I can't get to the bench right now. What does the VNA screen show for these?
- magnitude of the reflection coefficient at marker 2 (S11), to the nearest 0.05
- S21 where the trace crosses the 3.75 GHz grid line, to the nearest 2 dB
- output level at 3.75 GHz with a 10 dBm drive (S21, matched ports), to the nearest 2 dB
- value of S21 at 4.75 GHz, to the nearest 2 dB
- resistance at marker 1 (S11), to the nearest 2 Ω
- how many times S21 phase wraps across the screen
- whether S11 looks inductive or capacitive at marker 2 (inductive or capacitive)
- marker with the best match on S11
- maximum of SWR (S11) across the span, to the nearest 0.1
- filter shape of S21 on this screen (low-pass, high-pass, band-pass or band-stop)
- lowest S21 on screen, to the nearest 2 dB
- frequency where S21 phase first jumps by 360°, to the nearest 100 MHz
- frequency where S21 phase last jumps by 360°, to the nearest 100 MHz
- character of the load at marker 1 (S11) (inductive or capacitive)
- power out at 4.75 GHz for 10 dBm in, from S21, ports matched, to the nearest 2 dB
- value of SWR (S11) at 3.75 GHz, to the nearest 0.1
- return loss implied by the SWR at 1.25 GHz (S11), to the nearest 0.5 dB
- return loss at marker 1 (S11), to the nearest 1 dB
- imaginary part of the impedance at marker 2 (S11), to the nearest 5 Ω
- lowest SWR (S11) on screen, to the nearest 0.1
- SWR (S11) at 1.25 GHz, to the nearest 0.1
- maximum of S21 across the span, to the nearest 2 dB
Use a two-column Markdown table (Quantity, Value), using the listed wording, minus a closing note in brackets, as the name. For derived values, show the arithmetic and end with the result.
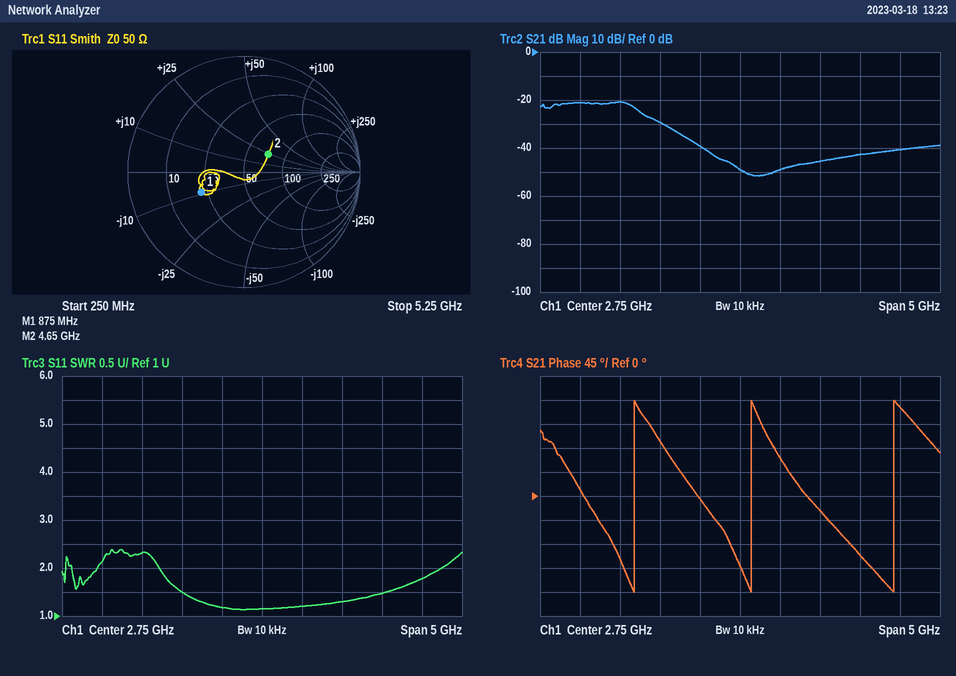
| Quantity | Value |
|---|---|
| magnitude of the reflection coefficient at marker 2 (S11), to the nearest 0.05 | 0.25 |
| S21 where the trace crosses the 3.75 GHz grid line, to the nearest 2 dB | -46 dB |
| output level at 3.75 GHz with a 10 dBm drive (S21, matched ports), to the nearest 2 dB | 10 dBm + (-46 dB) = -36 dBm |
| value of S21 at 4.75 GHz, to the nearest 2 dB | -40 dB |
| resistance at marker 1 (S11), to the nearest 2 Ω | 22 Ω |
| how many times S21 phase wraps across the screen | 3 |
| whether S11 looks inductive or capacitive at marker 2 | inductive |
| marker with the best match on S11 | marker 2 |
| maximum of SWR (S11) across the span, to the nearest 0.1 | 2.4 |
| filter shape of S21 on this screen | low-pass |
| lowest S21 on screen, to the nearest 2 dB | -52 dB |
| frequency where S21 phase first jumps by 360°, to the nearest 100 MHz | 1.4 GHz |
| frequency where S21 phase last jumps by 360°, to the nearest 100 MHz | 4.7 GHz |
| character of the load at marker 1 (S11) | capacitive |
| power out at 4.75 GHz for 10 dBm in, from S21, ports matched, to the nearest 2 dB | 10 dBm + (-40 dB) = -30 dBm |
| value of SWR (S11) at 3.75 GHz, to the nearest 0.1 | 1.3 |
| return loss implied by the SWR at 1.25 GHz (S11), to the nearest 0.5 dB | −20 log10((2.3 − 1)/(2.3 + 1)) ≈ 8.09 dB, so 8.0 dB to the nearest 0.5 dB |
| return loss at marker 1 (S11), to the nearest 1 dB | 8 dB |
| imaginary part of the impedance at marker 2 (S11), to the nearest 5 Ω | +25 Ω |
| lowest SWR (S11) on screen, to the nearest 0.1 | 1.1 |
| SWR (S11) at 1.25 GHz, to the nearest 0.1 | 2.3 |
| maximum of S21 across the span, to the nearest 2 dB | -20 dB |
